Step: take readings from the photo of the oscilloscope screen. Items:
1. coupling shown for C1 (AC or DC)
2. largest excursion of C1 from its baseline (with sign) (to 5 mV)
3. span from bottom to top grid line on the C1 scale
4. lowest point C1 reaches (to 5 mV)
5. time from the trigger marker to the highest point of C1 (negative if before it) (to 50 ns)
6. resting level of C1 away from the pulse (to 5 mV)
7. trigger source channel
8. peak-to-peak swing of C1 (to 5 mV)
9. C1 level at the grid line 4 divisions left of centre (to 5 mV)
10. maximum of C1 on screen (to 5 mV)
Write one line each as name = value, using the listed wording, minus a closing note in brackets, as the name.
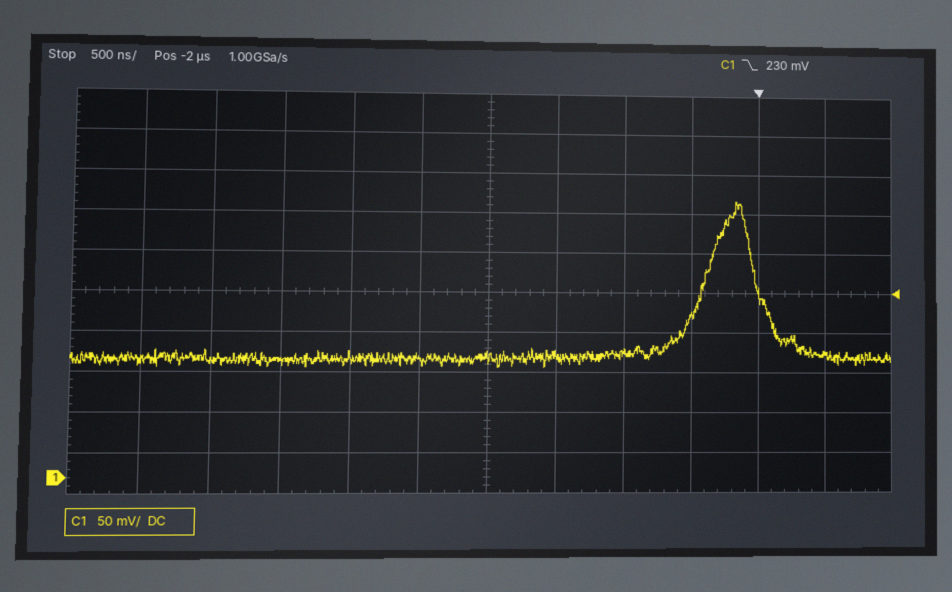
coupling shown for C1 = DC
largest excursion of C1 from its baseline (with sign) = +200 mV
span from bottom to top grid line on the C1 scale = 500 mV
lowest point C1 reaches = 135 mV
time from the trigger marker to the highest point of C1 (negative if before it) = -150 ns
resting level of C1 away from the pulse = 145 mV
trigger source channel = C1
peak-to-peak swing of C1 = 210 mV
C1 level at the grid line 4 divisions left of centre = 145 mV
maximum of C1 on screen = 345 mV
